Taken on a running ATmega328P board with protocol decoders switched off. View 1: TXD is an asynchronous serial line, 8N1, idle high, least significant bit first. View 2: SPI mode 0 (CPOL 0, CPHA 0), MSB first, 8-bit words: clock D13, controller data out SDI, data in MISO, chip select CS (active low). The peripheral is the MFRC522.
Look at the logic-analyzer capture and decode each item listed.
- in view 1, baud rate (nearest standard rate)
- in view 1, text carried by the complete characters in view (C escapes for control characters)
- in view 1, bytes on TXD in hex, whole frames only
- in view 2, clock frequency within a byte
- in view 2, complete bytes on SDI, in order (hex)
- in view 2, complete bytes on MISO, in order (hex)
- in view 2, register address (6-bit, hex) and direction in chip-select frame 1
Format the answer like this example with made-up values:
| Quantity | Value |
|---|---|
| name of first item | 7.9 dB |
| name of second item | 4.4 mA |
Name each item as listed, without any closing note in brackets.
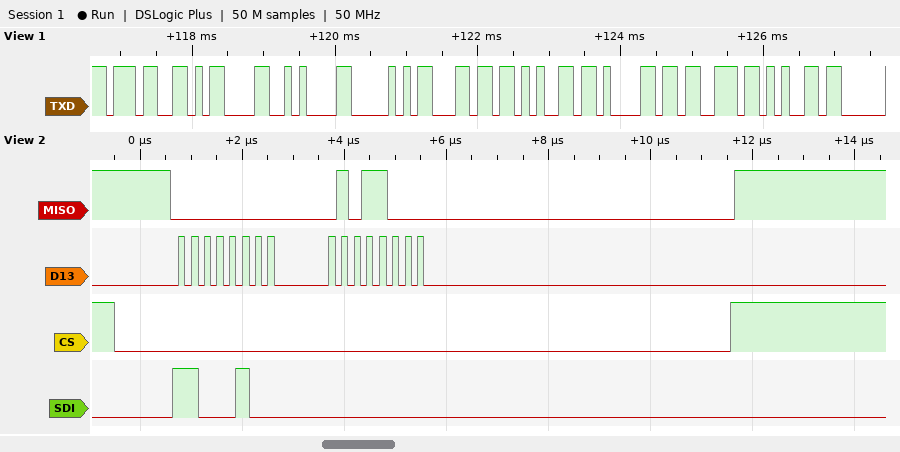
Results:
| Quantity | Value |
|---|---|
| in view 1, baud rate | 9600 baud |
| in view 1, text carried by the complete characters in view | "7\r\nPlease" |
| in view 1, bytes on TXD in hex, whole frames only | 0x37 0x0D 0x0A 0x50 0x6C 0x65 0x61 0x73 0x65 |
| in view 2, clock frequency within a byte | 4 MHz |
| in view 2, complete bytes on SDI, in order | C4 00 |
| in view 2, complete bytes on MISO, in order | 00 58 |
| in view 2, register address (6-bit, hex) and direction in chip-select frame 1 | 0x22 read |
